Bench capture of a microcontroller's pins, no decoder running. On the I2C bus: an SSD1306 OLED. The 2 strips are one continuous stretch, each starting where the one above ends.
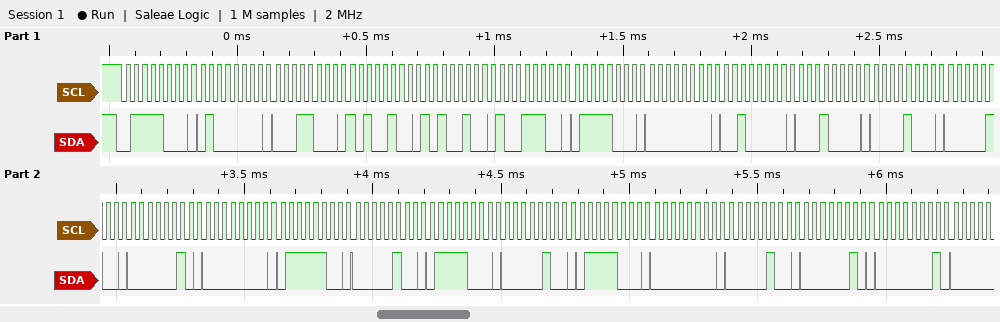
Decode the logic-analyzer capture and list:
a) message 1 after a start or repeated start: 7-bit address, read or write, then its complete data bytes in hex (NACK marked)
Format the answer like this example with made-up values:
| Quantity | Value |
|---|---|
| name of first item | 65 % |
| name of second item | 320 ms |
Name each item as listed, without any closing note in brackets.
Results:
| Quantity | Value |
|---|---|
| message 1 after a start or repeated start: 7-bit address, read or write, then its complete data bytes in hex | 0x3C write: 40 18 A4 A4 9C 78 00 20 10 08 04 02 00 7C 04 78 04 78 00 04 02 01 |
